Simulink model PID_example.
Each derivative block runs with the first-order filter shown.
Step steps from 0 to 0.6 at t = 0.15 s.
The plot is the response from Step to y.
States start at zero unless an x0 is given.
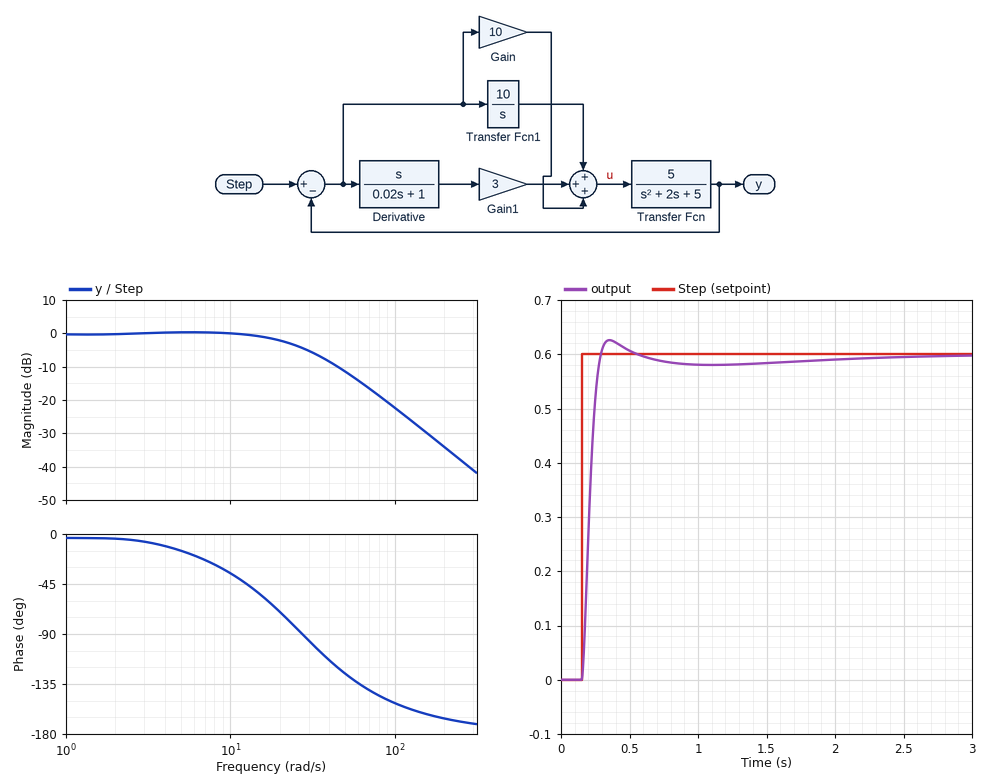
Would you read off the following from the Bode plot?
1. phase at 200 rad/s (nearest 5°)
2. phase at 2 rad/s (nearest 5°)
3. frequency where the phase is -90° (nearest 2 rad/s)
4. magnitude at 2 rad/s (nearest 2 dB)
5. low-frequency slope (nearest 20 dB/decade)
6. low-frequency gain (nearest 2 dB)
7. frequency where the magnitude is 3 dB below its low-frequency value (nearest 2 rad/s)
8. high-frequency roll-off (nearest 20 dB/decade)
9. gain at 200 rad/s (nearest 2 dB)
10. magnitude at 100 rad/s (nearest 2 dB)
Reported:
-165°
-5°
28 rad/s
0 dB
0 dB/decade
0 dB
24 rad/s
-40 dB/decade
-34 dB
-22 dB
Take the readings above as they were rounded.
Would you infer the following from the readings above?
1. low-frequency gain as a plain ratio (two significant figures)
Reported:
1.0
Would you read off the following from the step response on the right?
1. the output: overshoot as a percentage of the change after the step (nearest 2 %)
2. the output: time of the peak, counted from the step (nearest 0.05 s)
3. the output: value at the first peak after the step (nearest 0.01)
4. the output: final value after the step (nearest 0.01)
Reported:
4 %
0.20 s
0.63
0.60
